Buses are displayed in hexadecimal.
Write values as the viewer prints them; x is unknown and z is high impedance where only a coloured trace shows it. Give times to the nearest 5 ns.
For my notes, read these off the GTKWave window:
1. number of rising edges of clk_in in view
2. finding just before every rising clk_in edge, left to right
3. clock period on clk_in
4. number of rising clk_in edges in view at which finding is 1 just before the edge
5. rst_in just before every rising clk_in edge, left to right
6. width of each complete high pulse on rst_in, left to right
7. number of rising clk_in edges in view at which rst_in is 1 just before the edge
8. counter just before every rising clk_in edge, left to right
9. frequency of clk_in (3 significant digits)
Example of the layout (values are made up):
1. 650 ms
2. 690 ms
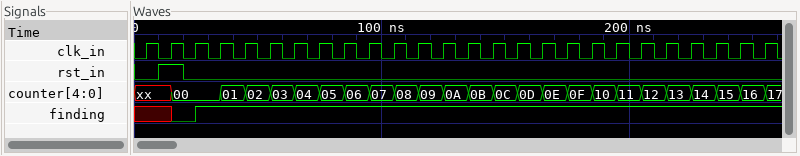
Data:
1. 26
2. x x 0 1 1 1 1 1 1 1 1 1 1 1 1 1 1 1 1 1 1 1 1 1 1 1
3. 10 ns
4. 23
5. 0 1 0 0 0 0 0 0 0 0 0 0 0 0 0 0 0 0 0 0 0 0 0 0 0 0
6. 10 ns
7. 1
8. xx, xx, 00, 00, 01, 02, 03, 04, 05, 06, 07, 08, 09, 0A, 0B, 0C, 0D, 0E, 0F, 10, 11, 12, 13, 14, 15, 16
9. 100 MHz
